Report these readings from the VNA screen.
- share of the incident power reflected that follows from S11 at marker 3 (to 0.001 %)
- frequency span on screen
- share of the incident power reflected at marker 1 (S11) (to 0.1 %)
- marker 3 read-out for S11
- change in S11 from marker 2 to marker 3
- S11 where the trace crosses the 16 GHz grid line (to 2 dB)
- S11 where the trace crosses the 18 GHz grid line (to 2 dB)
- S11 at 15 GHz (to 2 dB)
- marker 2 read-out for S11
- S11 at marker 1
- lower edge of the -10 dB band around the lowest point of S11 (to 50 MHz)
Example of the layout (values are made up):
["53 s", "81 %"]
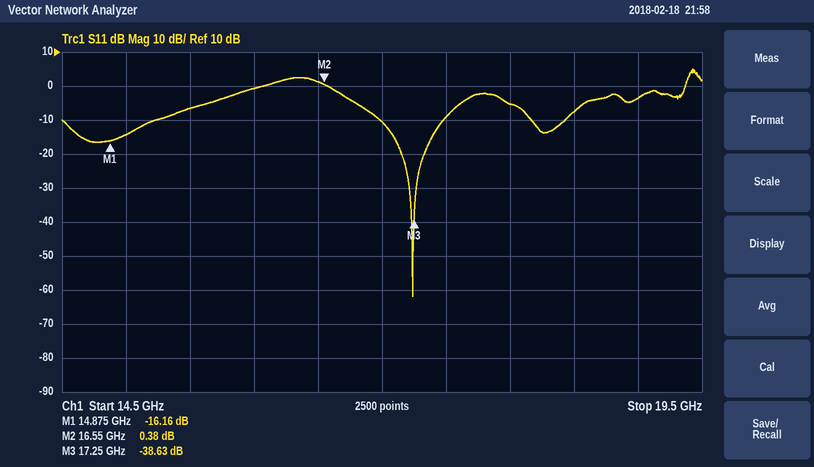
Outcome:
["0.014 %", "5 GHz", "2.4 %", "-38.63 dB", "-39.01 dB", "0 dB", "-6 dB", "-14 dB", "0.38 dB", "-16.16 dB", "17.00 GHz"]
